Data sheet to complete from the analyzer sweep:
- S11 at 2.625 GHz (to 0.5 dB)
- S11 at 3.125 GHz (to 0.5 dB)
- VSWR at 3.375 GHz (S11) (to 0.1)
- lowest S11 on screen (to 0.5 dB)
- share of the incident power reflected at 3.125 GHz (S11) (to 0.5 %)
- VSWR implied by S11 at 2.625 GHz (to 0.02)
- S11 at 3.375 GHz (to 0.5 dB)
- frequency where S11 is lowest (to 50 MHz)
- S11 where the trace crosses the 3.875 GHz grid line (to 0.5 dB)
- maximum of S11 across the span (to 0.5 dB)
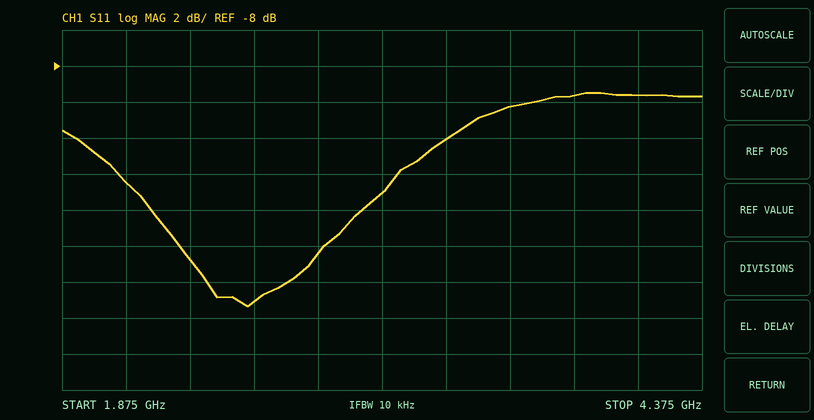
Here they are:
-21.0 dB
-15.0 dB
1.7
-21.5 dB
3.0 %
1.20
-12.0 dB
2.60 GHz
-9.5 dB
-9.5 dB
